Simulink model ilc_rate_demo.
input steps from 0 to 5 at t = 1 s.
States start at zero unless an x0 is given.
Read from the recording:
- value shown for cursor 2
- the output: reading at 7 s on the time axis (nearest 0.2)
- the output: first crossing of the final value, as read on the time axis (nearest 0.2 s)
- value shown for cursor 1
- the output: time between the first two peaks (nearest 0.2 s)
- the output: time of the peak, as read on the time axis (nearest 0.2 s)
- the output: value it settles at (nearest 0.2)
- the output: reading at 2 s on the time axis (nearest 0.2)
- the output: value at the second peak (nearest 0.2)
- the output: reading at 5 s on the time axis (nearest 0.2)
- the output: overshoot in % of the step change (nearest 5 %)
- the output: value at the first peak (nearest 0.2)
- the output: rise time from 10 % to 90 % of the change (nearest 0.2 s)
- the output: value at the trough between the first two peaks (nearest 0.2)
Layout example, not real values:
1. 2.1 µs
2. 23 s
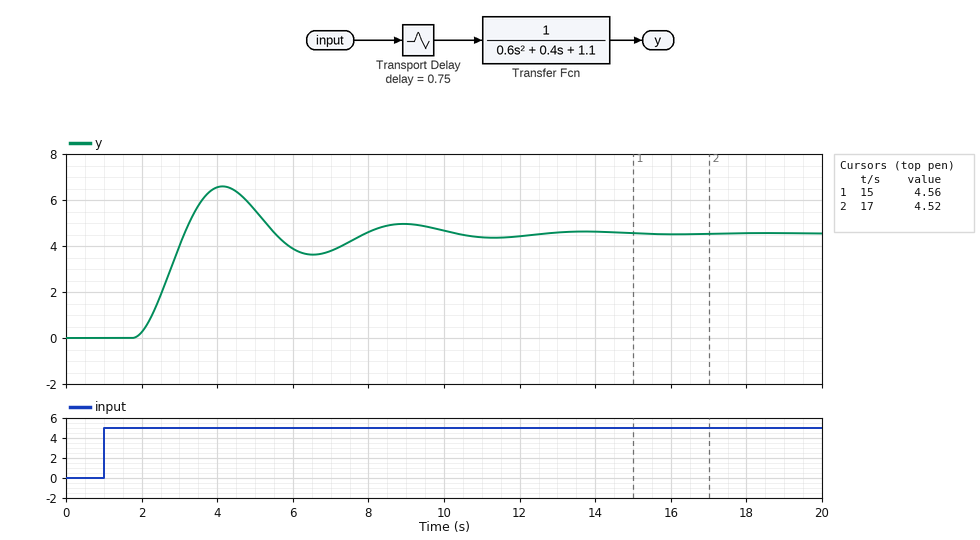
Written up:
1. 4.52
2. 3.8
3. 3.2 s
4. 4.56
5. 4.8 s
6. 4.2 s
7. 4.6
8. 0.2
9. 5.0
10. 5.6
11. 45 %
12. 6.6
13. 1.0 s
14. 3.6
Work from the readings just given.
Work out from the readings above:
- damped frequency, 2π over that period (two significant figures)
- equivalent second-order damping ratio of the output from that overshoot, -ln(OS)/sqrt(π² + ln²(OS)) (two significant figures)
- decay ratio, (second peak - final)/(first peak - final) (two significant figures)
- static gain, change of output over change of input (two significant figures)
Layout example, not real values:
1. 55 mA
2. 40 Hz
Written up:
1. 1.3 rad/s
2. 0.25
3. 0.20
4. 0.92
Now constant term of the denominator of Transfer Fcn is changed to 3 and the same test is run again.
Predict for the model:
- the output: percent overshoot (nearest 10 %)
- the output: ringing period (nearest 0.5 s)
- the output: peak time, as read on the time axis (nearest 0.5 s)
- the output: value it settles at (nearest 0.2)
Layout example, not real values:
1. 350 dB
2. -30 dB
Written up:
1. 60 %
2. 3.0 s
3. 3.0 s
4. 1.6
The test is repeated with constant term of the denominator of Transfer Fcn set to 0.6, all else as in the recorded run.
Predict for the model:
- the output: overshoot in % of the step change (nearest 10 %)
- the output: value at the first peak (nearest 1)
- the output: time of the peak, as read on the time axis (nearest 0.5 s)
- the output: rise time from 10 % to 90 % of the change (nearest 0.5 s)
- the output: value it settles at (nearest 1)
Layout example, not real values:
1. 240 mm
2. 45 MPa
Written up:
1. 30 %
2. 11
3. 5.0 s
4. 1.5 s
5. 8
